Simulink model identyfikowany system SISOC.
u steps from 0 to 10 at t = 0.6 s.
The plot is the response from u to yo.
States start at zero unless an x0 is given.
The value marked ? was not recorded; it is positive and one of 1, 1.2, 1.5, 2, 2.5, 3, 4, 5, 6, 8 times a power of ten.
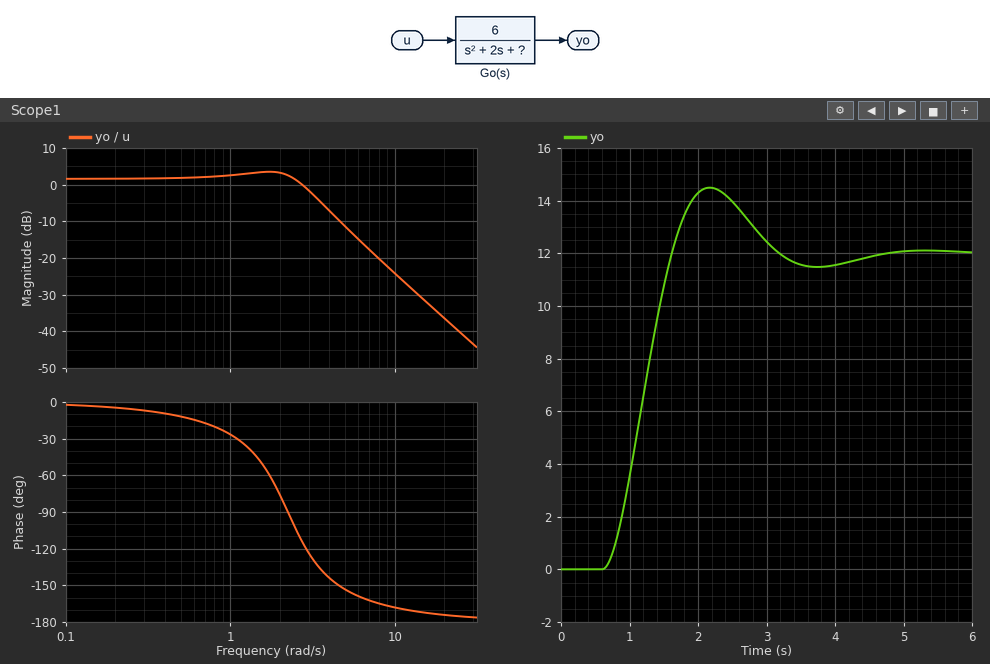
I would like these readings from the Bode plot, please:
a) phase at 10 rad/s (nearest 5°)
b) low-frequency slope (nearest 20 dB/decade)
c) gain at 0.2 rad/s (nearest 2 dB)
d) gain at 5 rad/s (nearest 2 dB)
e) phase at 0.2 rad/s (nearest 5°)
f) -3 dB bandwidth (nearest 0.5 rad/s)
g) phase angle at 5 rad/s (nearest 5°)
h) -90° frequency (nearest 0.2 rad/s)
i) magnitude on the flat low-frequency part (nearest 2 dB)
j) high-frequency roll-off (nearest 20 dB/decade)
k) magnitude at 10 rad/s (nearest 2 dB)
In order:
-170°
0 dB/decade
2 dB
-12 dB
-5°
3.0 rad/s
-155°
2.2 rad/s
2 dB
-40 dB/decade
-24 dB
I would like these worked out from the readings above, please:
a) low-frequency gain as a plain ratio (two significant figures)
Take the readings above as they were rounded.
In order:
1.3
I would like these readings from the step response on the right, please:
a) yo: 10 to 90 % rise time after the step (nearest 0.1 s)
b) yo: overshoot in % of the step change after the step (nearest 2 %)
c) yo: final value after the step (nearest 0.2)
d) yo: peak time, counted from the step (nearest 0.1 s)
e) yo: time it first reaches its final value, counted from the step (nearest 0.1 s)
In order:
0.7 s
20 %
12.0
1.6 s
1.0 s
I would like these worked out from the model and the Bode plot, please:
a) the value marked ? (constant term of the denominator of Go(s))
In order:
5
